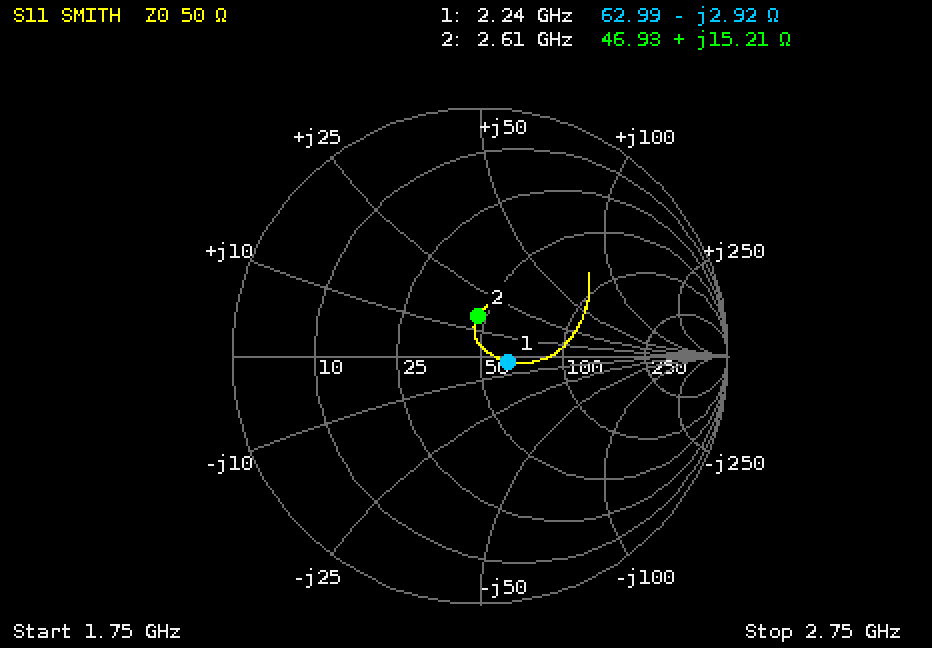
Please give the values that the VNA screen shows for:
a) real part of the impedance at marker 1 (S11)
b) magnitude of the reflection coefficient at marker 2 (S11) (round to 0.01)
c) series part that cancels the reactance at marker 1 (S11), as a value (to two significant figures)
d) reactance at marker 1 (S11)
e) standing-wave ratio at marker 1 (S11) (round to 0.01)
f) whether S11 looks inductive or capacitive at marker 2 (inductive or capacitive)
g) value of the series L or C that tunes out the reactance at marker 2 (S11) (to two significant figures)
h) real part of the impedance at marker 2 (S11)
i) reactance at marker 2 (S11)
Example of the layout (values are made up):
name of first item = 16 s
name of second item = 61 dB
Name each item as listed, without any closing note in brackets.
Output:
real part of the impedance at marker 1 = 62.99 Ω
magnitude of the reflection coefficient at marker 2 (S11) = 0.16
series part that cancels the reactance at marker 1 (S11), as a value = 210 pH
reactance at marker 1 = -2.92 Ω
standing-wave ratio at marker 1 (S11) = 1.27
whether S11 looks inductive or capacitive at marker 2 = inductive
value of the series L or C that tunes out the reactance at marker 2 (S11) = 4.0 pF
real part of the impedance at marker 2 = 46.93 Ω
reactance at marker 2 = +15.21 Ω
